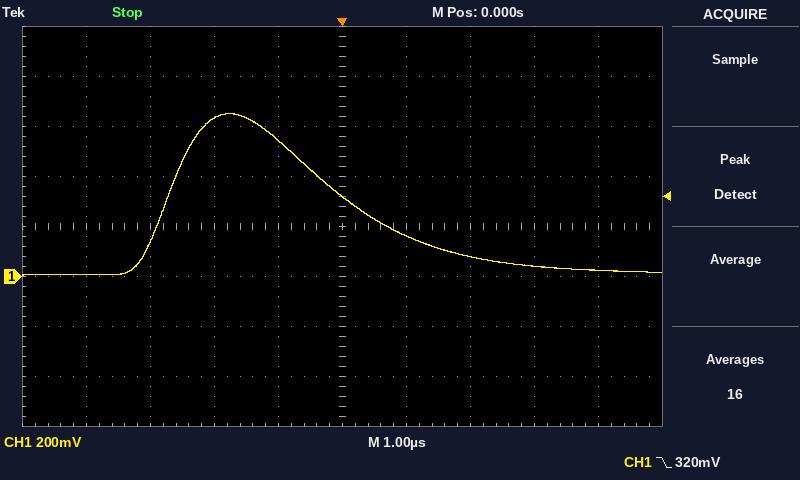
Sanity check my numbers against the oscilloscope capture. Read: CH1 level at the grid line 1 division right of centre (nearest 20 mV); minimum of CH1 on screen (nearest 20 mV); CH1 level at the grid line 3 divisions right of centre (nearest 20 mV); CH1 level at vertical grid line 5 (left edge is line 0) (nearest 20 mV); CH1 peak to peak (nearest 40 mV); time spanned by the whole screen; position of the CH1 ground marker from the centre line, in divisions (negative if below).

160 mV
0 mV
40 mV
320 mV
640 mV
10 µs
-1.0 div
